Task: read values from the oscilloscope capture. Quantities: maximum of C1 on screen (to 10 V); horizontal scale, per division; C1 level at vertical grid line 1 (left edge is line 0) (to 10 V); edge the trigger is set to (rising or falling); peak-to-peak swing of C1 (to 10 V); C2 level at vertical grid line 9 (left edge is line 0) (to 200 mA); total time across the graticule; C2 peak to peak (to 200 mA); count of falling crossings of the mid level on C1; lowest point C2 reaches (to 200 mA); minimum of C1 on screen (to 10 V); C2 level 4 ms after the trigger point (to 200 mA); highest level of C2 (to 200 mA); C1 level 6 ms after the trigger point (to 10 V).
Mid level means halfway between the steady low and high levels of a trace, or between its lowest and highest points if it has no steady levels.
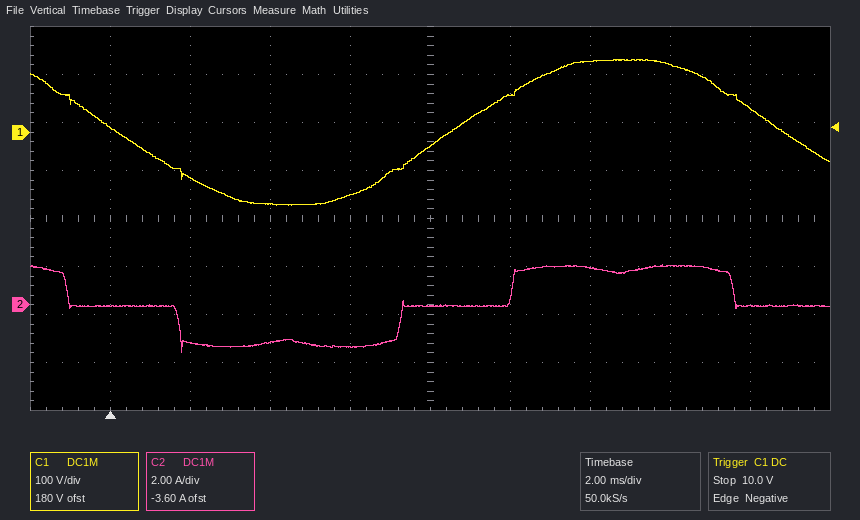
150 V
2 ms
10 V
falling
300 V
0.0 A
20 ms
3.6 A
2
-2.0 A
-150 V
-1.6 A
1.6 A
-130 V
